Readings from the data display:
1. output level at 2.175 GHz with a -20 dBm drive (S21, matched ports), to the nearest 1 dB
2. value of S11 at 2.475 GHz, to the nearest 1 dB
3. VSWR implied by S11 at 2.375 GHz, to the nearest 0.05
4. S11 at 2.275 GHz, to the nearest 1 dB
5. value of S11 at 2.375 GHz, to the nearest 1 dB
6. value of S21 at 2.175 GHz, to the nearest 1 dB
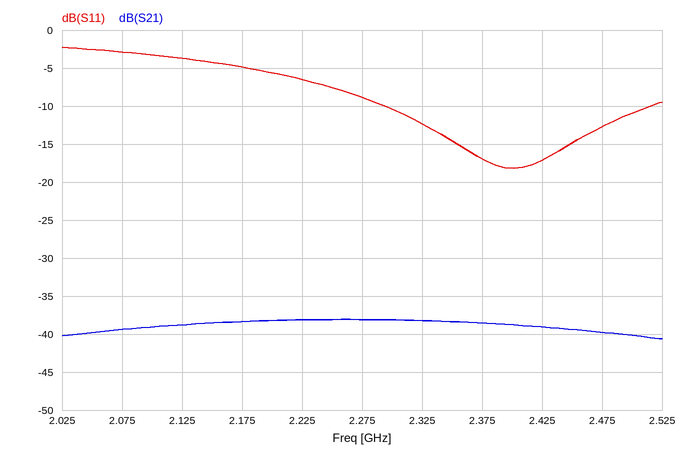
-58 dBm
-13 dB
1.35
-9 dB
-17 dB
-38 dB
